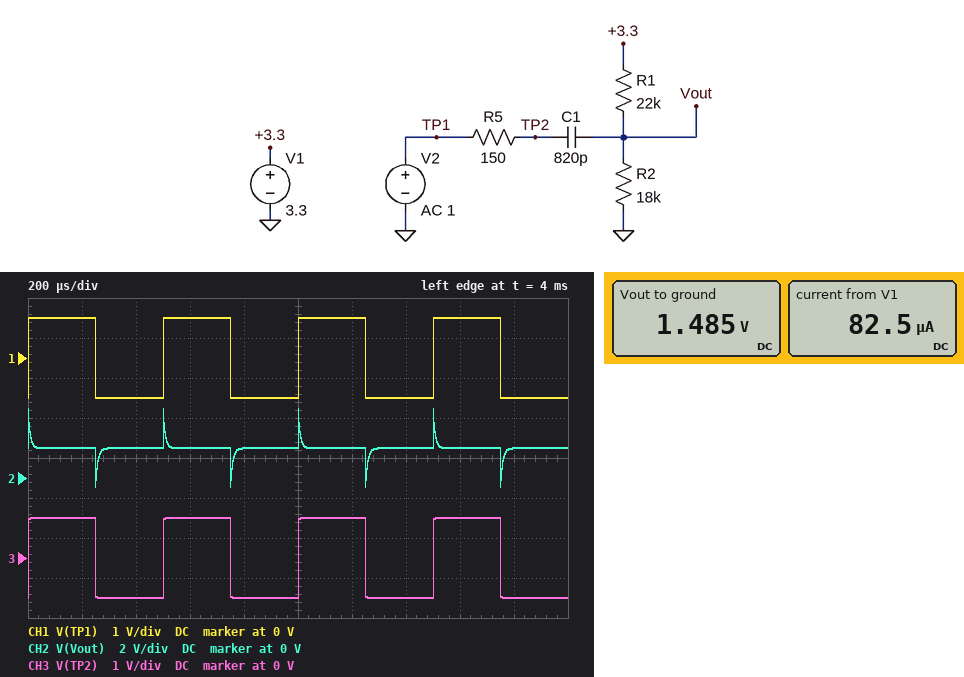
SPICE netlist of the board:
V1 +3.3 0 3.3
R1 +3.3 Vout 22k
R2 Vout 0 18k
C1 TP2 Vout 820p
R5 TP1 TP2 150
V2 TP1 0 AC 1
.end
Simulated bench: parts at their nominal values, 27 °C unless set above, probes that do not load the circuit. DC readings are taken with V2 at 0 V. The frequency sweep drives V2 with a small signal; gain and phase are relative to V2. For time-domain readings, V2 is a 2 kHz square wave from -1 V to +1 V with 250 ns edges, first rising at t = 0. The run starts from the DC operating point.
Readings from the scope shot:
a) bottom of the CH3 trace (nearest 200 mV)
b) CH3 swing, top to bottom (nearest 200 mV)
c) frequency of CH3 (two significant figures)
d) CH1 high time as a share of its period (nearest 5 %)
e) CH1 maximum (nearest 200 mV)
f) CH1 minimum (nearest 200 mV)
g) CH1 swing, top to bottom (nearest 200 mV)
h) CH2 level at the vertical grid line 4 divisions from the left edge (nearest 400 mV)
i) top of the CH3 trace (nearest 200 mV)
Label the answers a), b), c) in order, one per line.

a) -1.0 V
b) 2.0 V
c) 2.0 kHz
d) 50 %
e) 1.0 V
f) -1.0 V
g) 2.0 V
h) 1.6 V
i) 1.0 V
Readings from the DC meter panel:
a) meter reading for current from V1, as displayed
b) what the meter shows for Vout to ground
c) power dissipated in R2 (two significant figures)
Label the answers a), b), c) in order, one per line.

a) 82.5 µA
b) 1.485 V
c) 120 µW
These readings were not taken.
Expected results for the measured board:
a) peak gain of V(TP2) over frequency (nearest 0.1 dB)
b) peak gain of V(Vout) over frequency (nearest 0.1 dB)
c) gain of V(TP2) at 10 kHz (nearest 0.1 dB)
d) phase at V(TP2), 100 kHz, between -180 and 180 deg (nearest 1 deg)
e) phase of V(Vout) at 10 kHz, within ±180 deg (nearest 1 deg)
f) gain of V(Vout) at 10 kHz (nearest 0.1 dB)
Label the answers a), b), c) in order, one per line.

a) 0 dB
b) -0.1 dB
c) 0 dB
d) 0 deg
e) 63 deg
f) -6.9 dB
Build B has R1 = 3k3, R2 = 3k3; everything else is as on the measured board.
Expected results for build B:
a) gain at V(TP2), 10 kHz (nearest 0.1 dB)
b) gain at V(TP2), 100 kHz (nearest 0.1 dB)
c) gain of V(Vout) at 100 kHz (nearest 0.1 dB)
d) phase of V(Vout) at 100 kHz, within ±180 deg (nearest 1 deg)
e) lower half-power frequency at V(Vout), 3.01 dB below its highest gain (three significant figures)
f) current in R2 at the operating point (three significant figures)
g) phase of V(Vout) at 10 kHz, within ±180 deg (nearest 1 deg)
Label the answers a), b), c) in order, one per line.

a) 0 dB
b) -0.3 dB
c) -4.1 dB
d) 47 deg
e) 108 kHz
f) 500 µA
g) 85 deg
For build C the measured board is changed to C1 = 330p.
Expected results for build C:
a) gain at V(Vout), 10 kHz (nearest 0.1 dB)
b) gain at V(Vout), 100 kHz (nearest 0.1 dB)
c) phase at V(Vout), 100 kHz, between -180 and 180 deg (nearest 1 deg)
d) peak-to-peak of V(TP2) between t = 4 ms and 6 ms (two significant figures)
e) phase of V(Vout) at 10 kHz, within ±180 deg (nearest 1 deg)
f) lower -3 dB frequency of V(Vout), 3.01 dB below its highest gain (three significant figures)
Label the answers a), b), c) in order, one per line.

a) -13.9 dB
b) -1.0 dB
c) 26 deg
d) 2.0 V
e) 78 deg
f) 48.0 kHz
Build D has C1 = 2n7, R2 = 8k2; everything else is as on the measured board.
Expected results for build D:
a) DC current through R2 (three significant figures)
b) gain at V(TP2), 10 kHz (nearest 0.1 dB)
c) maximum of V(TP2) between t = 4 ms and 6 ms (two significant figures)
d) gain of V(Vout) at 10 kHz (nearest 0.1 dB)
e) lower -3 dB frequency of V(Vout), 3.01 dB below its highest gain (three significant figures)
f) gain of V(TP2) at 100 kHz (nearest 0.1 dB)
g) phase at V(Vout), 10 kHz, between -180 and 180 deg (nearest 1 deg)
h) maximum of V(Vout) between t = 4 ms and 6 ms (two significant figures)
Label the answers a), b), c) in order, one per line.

a) 109 µA
b) -0.1 dB
c) 1.0 V
d) -3.1 dB
e) 9.63 kHz
f) -0.2 dB
g) 44 deg
h) 2.8 V
